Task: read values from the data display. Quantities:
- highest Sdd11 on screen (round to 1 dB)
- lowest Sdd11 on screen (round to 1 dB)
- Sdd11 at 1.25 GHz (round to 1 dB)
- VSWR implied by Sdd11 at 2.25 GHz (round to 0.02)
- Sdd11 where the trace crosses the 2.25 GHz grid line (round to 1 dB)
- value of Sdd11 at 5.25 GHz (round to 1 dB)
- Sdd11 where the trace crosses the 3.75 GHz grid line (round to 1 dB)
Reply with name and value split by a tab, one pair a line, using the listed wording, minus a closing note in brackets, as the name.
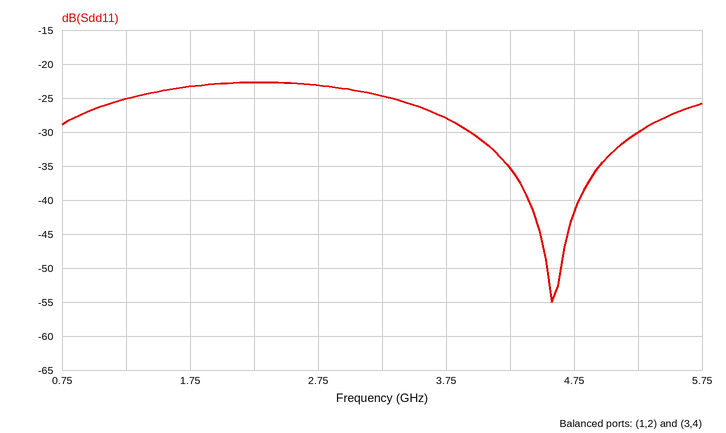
highest Sdd11 on screen	-23 dB
lowest Sdd11 on screen	-55 dB
Sdd11 at 1.25 GHz	-25 dB
VSWR implied by Sdd11 at 2.25 GHz	1.16
Sdd11 where the trace crosses the 2.25 GHz grid line	-23 dB
value of Sdd11 at 5.25 GHz	-30 dB
Sdd11 where the trace crosses the 3.75 GHz grid line	-28 dB
